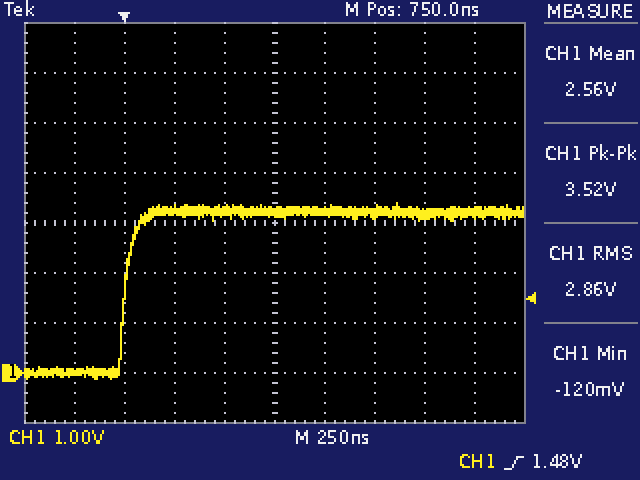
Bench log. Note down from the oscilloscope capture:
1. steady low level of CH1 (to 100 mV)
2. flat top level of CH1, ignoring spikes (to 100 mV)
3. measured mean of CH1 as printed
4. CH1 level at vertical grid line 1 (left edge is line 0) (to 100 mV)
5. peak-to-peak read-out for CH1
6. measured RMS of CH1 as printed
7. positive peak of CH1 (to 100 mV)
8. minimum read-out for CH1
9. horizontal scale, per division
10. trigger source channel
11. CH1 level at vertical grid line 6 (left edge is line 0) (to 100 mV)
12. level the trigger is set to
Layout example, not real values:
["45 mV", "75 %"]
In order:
["0.0 V", "3.2 V", "2.56 V", "0.0 V", "3.52 V", "2.86 V", "3.4 V", "-120 mV", "250 ns", "CH1", "3.2 V", "1.48 V"]
